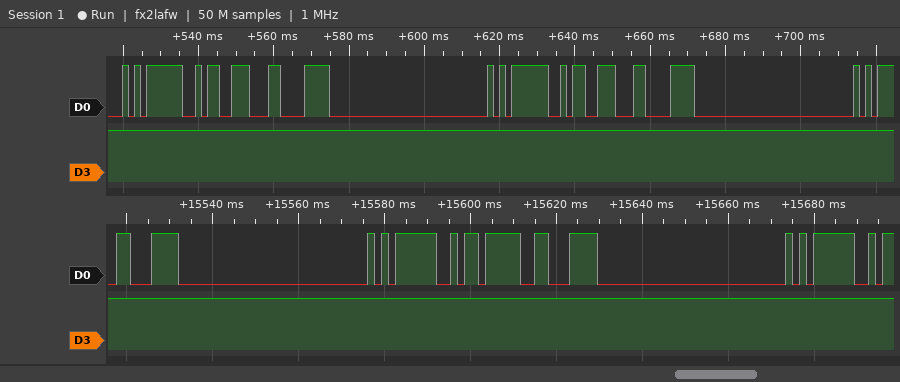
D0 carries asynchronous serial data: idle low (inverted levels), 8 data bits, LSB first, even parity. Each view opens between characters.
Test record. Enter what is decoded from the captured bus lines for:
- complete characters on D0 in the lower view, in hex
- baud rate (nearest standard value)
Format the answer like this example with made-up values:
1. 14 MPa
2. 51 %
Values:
1. 0E, 05, 09, 0E, 05
2. 600 baud
